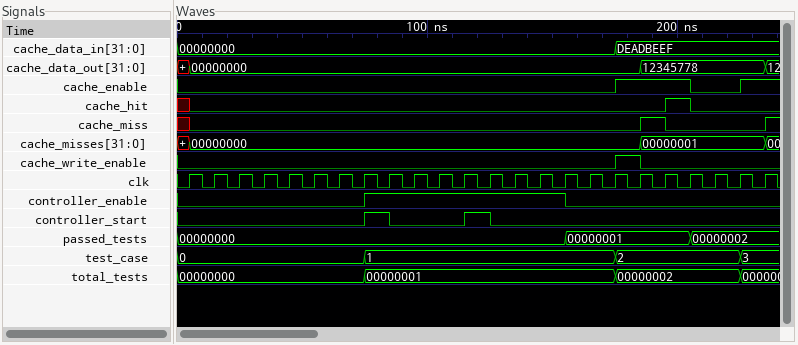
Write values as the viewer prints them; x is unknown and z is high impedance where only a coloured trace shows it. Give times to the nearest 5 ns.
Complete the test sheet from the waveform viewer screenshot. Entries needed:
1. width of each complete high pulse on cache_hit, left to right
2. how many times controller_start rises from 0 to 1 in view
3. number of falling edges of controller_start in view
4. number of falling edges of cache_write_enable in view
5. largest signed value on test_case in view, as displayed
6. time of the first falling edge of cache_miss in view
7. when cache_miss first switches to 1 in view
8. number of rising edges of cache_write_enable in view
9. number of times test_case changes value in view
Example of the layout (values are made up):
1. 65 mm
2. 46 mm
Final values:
1. 10 ns
2. 2
3. 2
4. 1
5. 3
6. 195 ns
7. 185 ns
8. 1
9. 3
